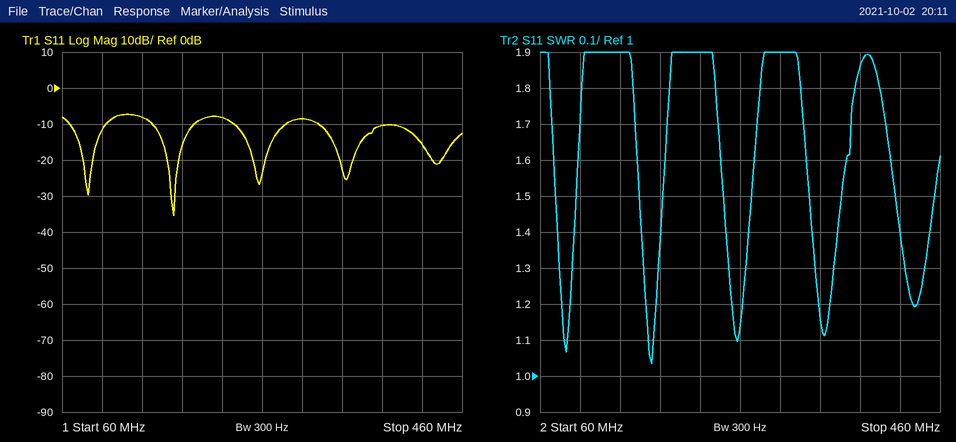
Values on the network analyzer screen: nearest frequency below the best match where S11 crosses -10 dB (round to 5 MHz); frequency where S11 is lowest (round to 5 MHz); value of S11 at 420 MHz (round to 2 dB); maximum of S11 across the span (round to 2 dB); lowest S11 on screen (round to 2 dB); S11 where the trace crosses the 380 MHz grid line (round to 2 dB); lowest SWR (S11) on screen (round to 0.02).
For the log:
150 MHz
170 MHz
-16 dB
-8 dB
-36 dB
-10 dB
1.04
